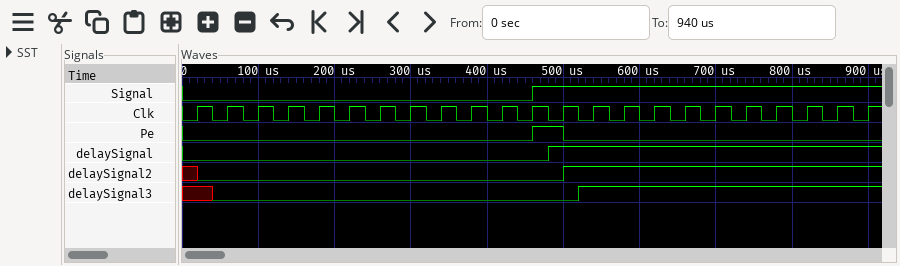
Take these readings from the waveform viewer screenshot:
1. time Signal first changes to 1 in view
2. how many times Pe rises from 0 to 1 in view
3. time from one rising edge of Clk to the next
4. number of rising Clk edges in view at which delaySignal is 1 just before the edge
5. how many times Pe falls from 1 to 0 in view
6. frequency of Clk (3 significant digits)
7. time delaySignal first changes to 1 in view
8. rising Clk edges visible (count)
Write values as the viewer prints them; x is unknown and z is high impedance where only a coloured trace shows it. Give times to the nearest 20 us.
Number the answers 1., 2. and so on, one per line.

1. 460 us
2. 1
3. 40 us
4. 11
5. 1
6. 25.0 kHz
7. 480 us
8. 23
